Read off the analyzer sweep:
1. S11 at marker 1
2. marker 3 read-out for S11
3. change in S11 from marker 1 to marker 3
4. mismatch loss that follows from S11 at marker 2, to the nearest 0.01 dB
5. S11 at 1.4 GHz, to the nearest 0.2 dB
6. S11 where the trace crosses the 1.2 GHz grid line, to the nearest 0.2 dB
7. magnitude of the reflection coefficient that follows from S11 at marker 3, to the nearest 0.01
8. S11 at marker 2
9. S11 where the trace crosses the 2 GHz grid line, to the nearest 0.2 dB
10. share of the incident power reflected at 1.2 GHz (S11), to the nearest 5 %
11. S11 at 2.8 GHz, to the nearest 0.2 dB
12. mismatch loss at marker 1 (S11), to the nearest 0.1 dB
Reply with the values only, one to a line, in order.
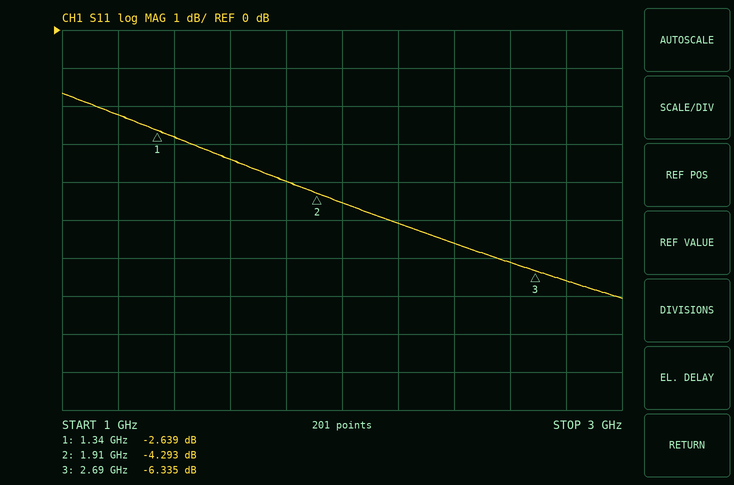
-2.639 dB
-6.335 dB
-3.696 dB
2.02 dB
-2.8 dB
-2.2 dB
0.48
-4.293 dB
-4.6 dB
60 %
-6.6 dB
3.4 dB
